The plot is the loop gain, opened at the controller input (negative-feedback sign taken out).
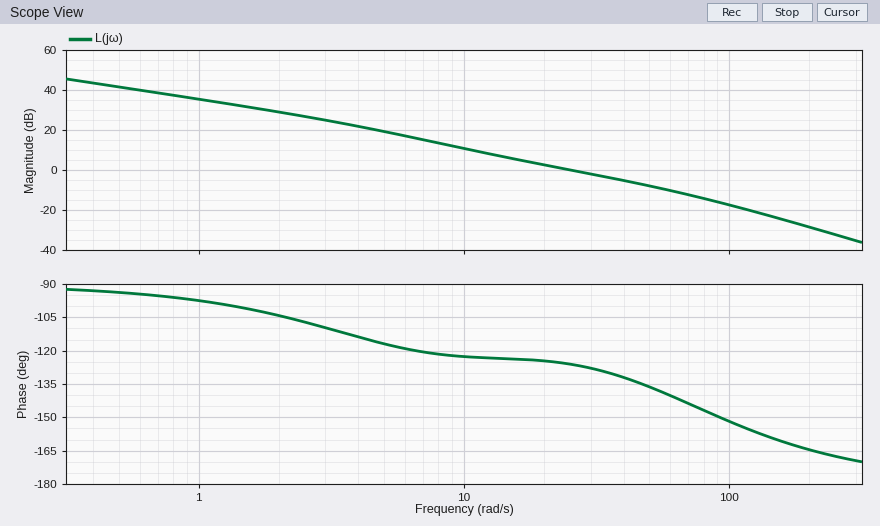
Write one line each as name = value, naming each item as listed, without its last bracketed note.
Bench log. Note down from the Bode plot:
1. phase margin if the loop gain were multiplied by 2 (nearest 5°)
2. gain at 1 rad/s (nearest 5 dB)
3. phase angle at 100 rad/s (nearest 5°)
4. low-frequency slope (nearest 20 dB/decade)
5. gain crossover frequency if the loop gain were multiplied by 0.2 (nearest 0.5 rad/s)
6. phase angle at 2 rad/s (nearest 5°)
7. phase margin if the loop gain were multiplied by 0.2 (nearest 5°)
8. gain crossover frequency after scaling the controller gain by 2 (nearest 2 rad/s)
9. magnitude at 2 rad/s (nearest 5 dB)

phase margin if the loop gain were multiplied by 2 = 45°
gain at 1 rad/s = 35 dB
phase angle at 100 rad/s = -150°
low-frequency slope = -20 dB/decade
gain crossover frequency if the loop gain were multiplied by 0.2 = 7.5 rad/s
phase angle at 2 rad/s = -105°
phase margin if the loop gain were multiplied by 0.2 = 60°
gain crossover frequency after scaling the controller gain by 2 = 42 rad/s
magnitude at 2 rad/s = 30 dB
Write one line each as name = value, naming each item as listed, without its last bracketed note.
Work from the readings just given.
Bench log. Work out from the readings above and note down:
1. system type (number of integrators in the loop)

system type = 1
